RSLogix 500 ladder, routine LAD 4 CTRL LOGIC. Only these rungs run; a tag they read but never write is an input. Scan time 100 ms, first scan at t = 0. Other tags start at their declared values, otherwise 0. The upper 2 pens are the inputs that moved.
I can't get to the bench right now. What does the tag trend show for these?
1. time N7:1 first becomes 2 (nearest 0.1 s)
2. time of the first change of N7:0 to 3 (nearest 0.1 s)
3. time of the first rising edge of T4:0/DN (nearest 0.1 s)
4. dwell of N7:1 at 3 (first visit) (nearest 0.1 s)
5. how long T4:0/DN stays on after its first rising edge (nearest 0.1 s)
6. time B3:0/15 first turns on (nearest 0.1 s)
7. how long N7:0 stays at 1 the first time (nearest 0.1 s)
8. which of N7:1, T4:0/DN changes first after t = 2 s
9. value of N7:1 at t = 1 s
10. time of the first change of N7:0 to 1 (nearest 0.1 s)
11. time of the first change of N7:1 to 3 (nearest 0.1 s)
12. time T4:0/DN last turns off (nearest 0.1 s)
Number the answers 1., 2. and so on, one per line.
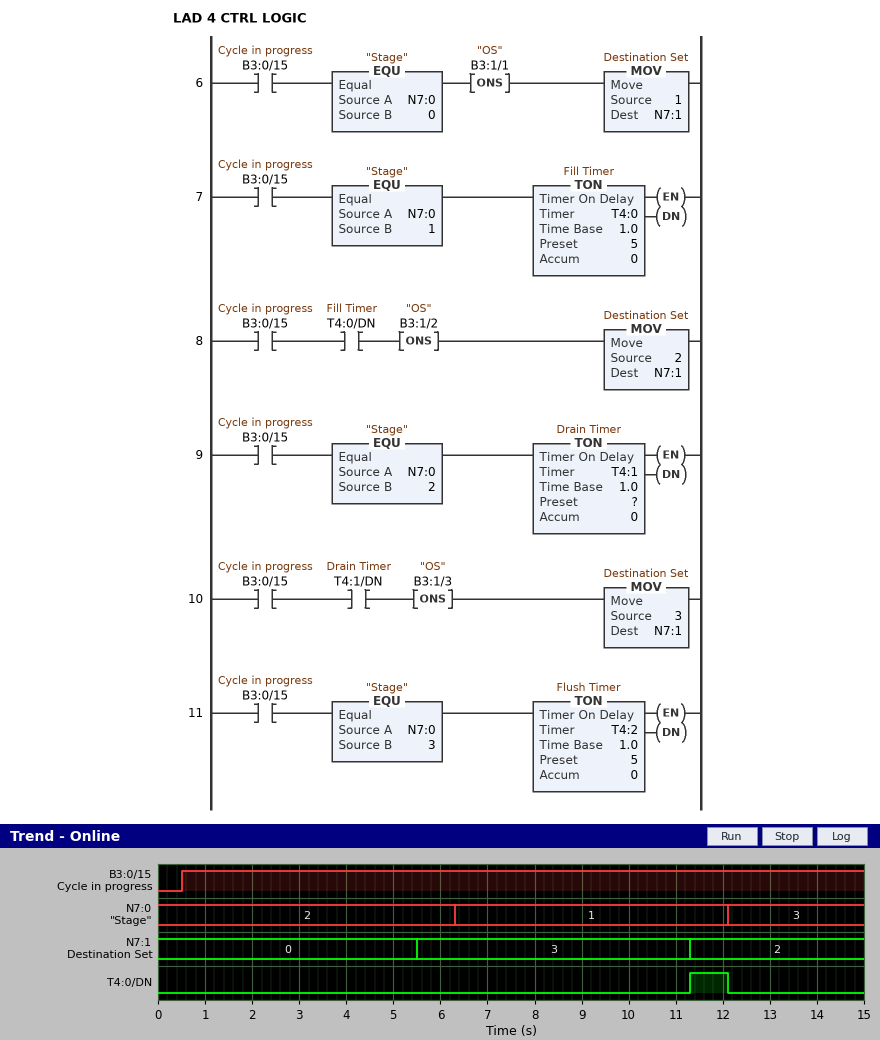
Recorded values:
1. 11.3 s
2. 12.1 s
3. 11.3 s
4. 5.8 s
5. 0.8 s
6. 0.5 s
7. 5.8 s
8. N7:1
9. 0
10. 6.3 s
11. 5.5 s
12. 12.1 s
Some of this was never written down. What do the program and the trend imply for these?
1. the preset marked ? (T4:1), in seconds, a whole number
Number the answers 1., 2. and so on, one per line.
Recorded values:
1. 5 s
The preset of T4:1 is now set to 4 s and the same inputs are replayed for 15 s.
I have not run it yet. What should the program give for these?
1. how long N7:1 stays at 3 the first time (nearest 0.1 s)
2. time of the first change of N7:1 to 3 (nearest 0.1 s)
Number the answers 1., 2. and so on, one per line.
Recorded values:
1. 6.8 s
2. 4.5 s
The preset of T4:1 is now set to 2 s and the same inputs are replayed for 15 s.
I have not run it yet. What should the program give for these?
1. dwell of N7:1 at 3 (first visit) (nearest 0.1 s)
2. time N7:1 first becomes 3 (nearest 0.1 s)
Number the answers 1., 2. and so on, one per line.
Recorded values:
1. 8.8 s
2. 2.5 s
